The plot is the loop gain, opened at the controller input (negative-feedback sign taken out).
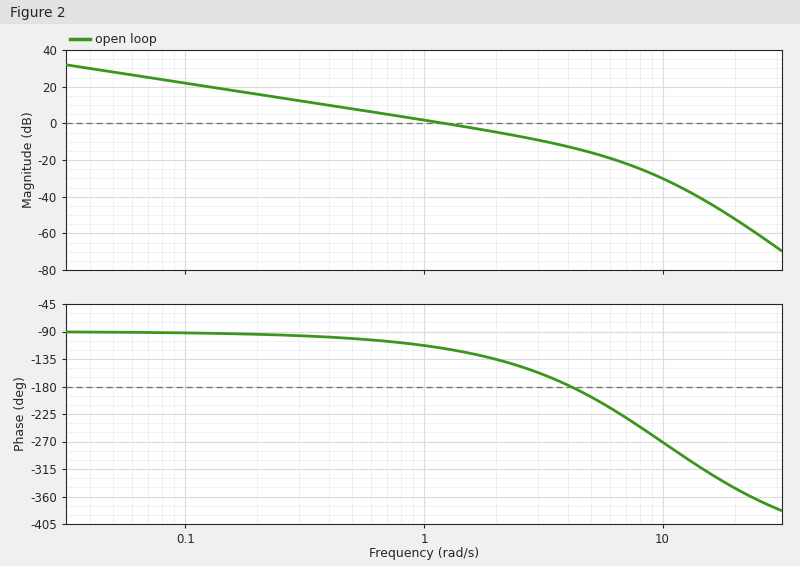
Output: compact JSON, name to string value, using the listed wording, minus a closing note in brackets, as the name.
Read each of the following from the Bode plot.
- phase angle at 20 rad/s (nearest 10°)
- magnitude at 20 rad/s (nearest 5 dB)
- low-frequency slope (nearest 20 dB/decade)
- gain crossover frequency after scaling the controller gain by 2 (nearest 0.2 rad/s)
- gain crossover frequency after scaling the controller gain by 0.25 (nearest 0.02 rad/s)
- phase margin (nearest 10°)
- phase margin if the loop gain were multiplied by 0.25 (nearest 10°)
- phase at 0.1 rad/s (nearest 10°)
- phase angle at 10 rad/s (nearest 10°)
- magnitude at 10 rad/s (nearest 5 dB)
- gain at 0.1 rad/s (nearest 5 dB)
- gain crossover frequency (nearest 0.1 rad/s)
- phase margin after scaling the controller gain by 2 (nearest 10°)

{"phase angle at 20 rad/s": "-350°", "magnitude at 20 rad/s": "-50 dB", "low-frequency slope": "-20 dB/decade", "gain crossover frequency after scaling the controller gain by 2": "2.2 rad/s", "gain crossover frequency after scaling the controller gain by 0.25": "0.32 rad/s", "phase margin": "60°", "phase margin if the loop gain were multiplied by 0.25": "80°", "phase at 0.1 rad/s": "-90°", "phase angle at 10 rad/s": "-270°", "magnitude at 10 rad/s": "-30 dB", "gain at 0.1 rad/s": "20 dB", "gain crossover frequency": "1.2 rad/s", "phase margin after scaling the controller gain by 2": "40°"}
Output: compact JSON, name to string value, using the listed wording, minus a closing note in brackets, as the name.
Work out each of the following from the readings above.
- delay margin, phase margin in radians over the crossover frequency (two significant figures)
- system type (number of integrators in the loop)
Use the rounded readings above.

{"delay margin, phase margin in radians over the crossover frequency": "0.87 s", "system type": "1"}
